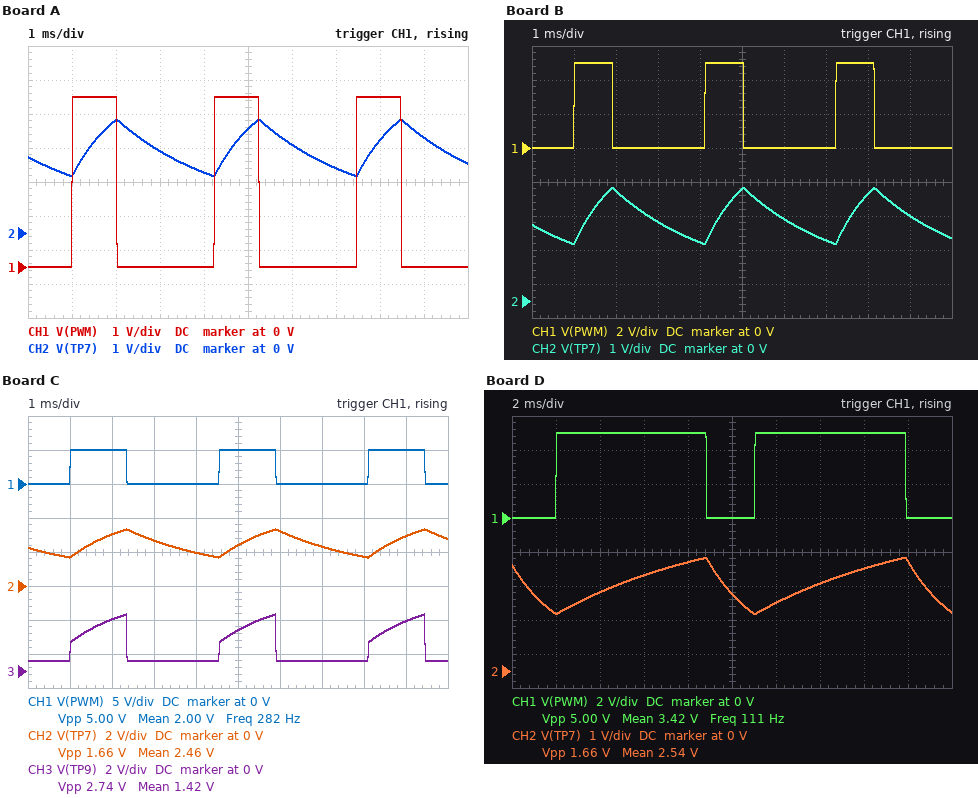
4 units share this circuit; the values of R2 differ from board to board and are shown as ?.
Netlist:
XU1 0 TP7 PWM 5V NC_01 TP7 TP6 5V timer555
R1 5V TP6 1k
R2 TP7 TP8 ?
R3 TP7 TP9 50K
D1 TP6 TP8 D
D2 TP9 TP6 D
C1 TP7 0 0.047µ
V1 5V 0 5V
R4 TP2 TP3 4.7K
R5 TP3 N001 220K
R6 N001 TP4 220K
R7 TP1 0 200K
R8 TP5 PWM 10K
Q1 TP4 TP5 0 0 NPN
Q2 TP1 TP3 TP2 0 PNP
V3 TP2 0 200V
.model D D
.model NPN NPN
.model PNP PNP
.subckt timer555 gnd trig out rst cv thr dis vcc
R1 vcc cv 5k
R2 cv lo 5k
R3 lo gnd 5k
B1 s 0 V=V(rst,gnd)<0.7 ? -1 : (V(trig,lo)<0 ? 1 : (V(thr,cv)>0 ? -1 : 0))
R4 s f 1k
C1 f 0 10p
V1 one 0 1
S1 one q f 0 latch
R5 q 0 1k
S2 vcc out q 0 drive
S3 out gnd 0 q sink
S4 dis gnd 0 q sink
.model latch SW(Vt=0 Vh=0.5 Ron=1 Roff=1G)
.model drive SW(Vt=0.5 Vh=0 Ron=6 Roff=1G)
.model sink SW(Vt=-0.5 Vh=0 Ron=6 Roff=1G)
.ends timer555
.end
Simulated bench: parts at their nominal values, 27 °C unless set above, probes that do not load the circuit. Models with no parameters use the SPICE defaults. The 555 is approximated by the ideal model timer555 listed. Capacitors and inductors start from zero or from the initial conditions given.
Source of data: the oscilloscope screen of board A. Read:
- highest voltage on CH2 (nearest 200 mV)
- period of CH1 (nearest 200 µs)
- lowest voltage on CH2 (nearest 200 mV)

3.4 V
3.2 ms
1.6 V
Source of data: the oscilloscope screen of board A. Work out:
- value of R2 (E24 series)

22 kΩ
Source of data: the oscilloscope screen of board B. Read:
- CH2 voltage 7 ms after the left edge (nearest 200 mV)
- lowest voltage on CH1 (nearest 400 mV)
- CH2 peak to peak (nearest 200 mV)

1.8 V
0 V
1.6 V
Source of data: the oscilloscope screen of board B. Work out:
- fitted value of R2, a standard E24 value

20 kΩ
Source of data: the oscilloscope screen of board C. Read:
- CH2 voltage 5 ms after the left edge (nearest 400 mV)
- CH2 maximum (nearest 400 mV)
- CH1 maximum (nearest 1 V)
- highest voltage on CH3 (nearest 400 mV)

2.4 V
3.2 V
5 V
3.2 V
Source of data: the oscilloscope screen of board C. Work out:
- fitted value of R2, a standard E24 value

30 kΩ
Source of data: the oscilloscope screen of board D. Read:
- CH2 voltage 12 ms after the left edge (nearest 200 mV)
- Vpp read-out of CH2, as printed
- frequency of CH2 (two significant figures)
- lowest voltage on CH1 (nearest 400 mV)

2.0 V
1.66 V
110 Hz
0 V
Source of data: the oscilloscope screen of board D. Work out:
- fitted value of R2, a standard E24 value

160 kΩ
